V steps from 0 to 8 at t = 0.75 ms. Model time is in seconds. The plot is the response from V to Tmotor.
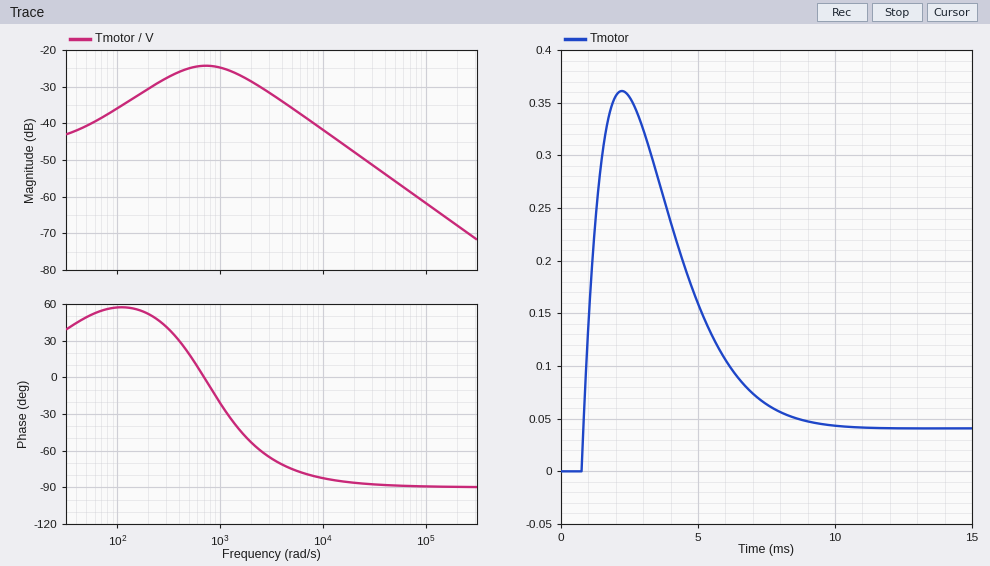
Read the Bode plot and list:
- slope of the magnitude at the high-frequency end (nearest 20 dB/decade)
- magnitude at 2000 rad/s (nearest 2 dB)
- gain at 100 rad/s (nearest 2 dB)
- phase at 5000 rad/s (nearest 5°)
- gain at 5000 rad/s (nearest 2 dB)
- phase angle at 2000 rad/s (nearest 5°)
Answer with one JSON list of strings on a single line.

["-20 dB/decade", "-28 dB", "-36 dB", "-75°", "-36 dB", "-55°"]
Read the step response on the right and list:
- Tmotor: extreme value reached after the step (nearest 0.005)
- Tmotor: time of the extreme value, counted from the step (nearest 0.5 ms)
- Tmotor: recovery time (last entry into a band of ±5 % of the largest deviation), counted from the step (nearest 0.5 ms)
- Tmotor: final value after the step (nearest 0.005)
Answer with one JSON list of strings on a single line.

["0.360", "1.5 ms", "7.0 ms", "0.040"]
